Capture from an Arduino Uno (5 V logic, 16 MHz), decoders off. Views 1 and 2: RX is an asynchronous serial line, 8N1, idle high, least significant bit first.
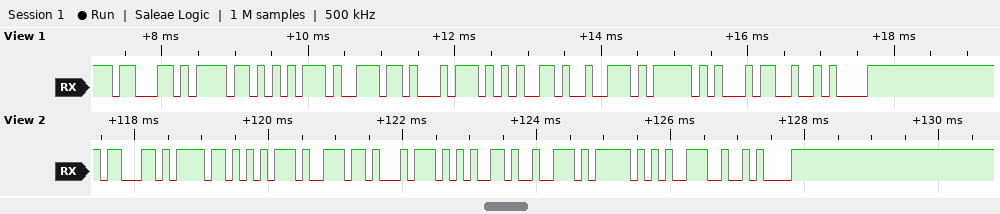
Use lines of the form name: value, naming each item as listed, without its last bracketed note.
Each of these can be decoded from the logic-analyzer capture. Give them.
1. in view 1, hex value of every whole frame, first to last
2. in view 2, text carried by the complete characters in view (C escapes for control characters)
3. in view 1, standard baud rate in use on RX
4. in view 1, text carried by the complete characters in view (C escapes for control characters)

in view 1, hex value of every whole frame, first to last: 0x63 0x6F 0x75 0x6E 0x74 0x65 0x72 0x5F 0x34 0x0A
in view 2, text carried by the complete characters in view: "counter_9\n"
in view 1, standard baud rate in use on RX: 9600 baud
in view 1, text carried by the complete characters in view: "counter_4\n"
